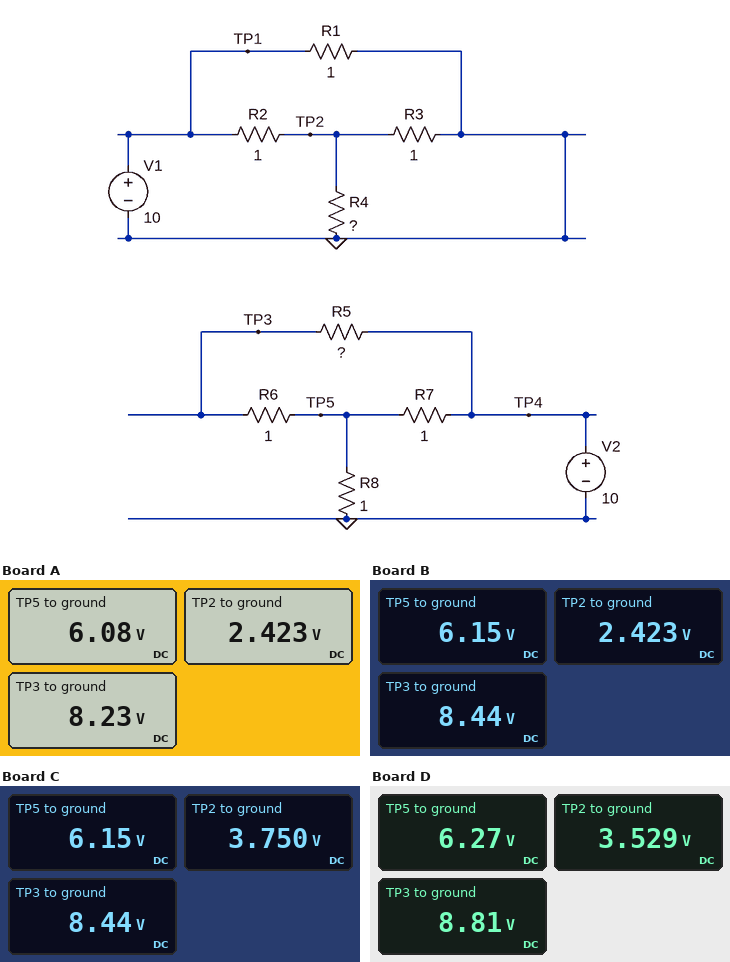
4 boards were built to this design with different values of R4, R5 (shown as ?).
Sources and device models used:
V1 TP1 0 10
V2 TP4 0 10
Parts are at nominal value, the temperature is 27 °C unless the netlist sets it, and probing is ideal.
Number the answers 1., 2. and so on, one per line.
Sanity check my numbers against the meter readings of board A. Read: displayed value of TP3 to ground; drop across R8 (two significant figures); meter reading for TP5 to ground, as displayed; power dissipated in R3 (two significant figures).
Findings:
1. 8.23 V
2. 6.1 V
3. 6.08 V
4. 5.9 W
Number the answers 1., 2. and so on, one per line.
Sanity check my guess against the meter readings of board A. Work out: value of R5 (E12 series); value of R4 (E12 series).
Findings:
1. 0.82 Ω
2. 0.47 Ω
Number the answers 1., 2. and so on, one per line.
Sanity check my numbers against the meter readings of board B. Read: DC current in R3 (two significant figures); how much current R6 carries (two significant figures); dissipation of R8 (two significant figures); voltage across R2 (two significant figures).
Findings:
1. 2.4 A
2. 2.3 A
3. 38 W
4. 7.6 V
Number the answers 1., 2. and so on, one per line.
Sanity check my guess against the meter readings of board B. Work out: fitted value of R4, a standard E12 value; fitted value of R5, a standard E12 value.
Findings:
1. 0.47 Ω
2. 0.68 Ω
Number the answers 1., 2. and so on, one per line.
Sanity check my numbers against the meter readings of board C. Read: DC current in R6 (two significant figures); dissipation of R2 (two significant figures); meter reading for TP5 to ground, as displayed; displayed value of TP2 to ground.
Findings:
1. 2.3 A
2. 39 W
3. 6.15 V
4. 3.750 V
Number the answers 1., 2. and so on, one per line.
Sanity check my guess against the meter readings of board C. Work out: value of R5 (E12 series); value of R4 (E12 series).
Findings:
1. 0.68 Ω
2. 1.5 Ω
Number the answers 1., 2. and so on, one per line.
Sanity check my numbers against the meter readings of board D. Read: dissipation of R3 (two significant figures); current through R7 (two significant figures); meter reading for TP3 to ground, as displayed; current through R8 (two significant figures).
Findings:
1. 12 W
2. 3.7 A
3. 8.81 V
4. 6.3 A
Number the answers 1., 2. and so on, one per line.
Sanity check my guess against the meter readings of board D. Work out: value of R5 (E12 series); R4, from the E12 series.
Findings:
1. 0.47 Ω
2. 1.2 Ω
